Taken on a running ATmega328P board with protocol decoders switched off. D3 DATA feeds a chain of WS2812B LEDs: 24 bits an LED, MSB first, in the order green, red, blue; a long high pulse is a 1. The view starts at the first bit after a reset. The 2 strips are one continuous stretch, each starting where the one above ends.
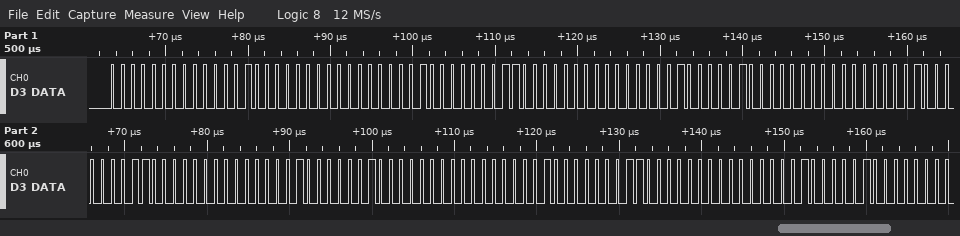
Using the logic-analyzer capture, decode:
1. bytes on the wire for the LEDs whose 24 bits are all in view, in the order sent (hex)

00 04 00 02 03 00 01 04 00 02 03 00 02 04 00 02 03 00
